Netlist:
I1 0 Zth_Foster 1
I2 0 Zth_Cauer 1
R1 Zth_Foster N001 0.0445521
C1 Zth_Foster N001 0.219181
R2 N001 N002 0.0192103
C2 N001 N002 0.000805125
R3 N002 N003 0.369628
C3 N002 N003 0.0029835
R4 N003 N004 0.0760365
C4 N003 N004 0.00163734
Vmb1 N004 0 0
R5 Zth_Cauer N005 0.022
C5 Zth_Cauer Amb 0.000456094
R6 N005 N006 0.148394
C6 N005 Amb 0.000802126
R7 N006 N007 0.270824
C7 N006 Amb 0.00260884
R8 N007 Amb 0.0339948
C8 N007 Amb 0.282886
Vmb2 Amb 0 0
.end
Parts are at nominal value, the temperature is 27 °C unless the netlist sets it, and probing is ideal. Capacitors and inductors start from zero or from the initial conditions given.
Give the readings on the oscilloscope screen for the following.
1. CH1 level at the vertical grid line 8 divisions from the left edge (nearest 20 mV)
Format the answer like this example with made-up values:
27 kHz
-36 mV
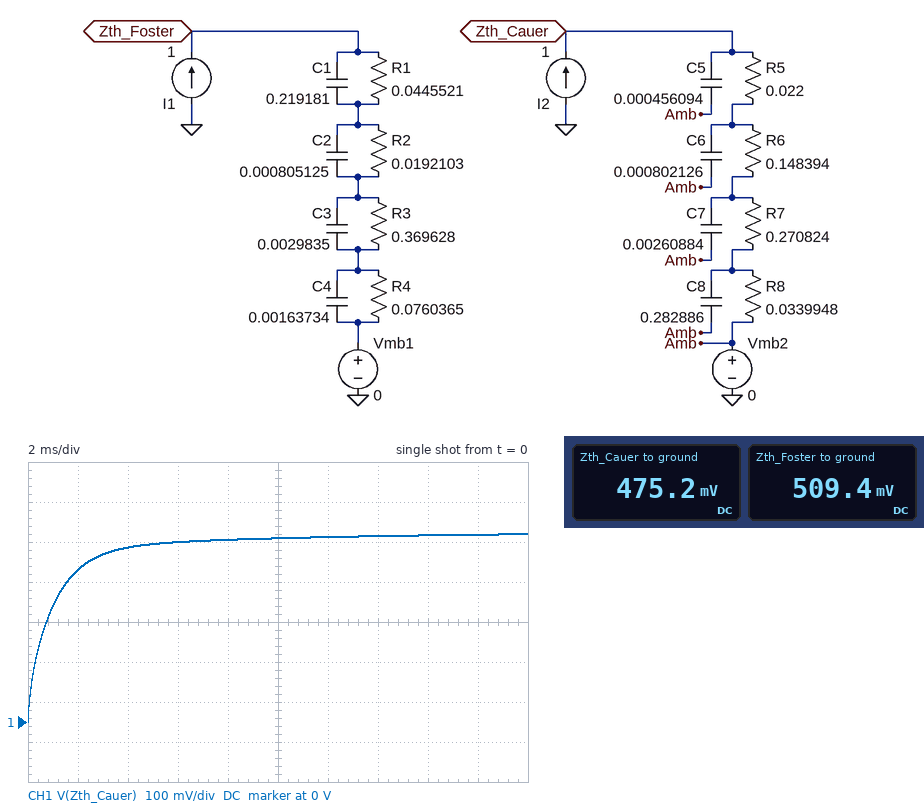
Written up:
460 mV
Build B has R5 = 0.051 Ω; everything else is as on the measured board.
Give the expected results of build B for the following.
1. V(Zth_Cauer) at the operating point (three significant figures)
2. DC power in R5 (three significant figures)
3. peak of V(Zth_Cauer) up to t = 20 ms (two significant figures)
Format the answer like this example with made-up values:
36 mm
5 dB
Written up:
504 mV
51.0 mW
500 mV
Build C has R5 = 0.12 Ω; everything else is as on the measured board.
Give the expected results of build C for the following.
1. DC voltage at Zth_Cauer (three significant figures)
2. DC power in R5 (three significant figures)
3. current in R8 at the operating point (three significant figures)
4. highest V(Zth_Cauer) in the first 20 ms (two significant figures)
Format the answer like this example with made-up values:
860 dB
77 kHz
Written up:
573 mV
120 mW
1.00 A
570 mV
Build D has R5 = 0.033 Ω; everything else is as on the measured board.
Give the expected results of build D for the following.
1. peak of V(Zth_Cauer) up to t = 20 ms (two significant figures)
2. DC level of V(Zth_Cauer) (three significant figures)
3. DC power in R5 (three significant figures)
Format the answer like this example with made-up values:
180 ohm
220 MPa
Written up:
480 mV
486 mV
33.0 mW
